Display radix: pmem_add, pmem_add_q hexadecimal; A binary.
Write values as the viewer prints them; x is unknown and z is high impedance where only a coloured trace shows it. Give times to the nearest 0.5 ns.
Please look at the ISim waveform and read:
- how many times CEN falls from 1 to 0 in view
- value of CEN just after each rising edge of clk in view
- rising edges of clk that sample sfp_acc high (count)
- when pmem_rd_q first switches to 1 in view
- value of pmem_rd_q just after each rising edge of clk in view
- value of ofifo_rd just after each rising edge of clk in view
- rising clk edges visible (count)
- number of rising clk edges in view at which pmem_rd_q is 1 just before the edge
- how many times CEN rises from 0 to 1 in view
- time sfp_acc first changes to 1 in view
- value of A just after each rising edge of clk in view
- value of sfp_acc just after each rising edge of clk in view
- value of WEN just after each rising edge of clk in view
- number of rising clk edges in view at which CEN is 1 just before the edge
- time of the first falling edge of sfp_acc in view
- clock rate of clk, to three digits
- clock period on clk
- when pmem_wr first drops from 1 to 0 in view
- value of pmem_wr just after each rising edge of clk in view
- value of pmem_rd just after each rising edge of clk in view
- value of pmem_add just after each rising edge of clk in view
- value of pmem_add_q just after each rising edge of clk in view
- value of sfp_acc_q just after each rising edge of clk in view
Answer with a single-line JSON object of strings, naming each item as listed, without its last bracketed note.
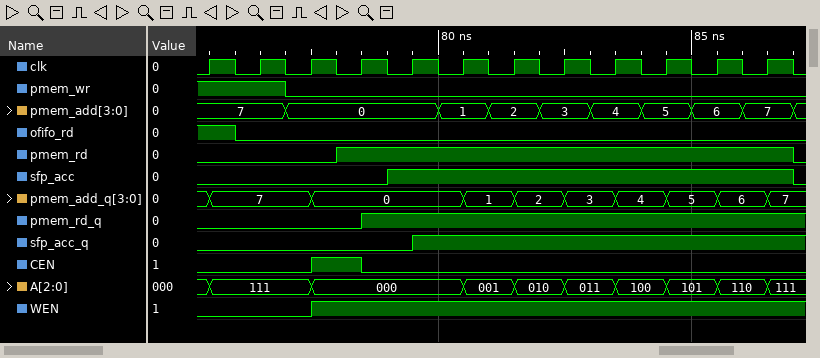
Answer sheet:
{"how many times CEN falls from 1 to 0 in view": "1", "value of CEN just after each rising edge of clk in view": "0 0 1 0 0 0 0 0 0 0 0 0", "rising edges of clk that sample sfp_acc high": "8", "when pmem_rd_q first switches to 1 in view": "78.5 ns", "value of pmem_rd_q just after each rising edge of clk in view": "0 0 0 1 1 1 1 1 1 1 1 1", "value of ofifo_rd just after each rising edge of clk in view": "1 0 0 0 0 0 0 0 0 0 0 0", "rising clk edges visible": "12", "number of rising clk edges in view at which pmem_rd_q is 1 just before the edge": "8", "how many times CEN rises from 0 to 1 in view": "1", "time sfp_acc first changes to 1 in view": "79 ns", "value of A just after each rising edge of clk in view": "111, 111, 000, 000, 000, 001, 010, 011, 100, 101, 110, 111", "value of sfp_acc just after each rising edge of clk in view": "0 0 0 0 1 1 1 1 1 1 1 1", "value of WEN just after each rising edge of clk in view": "0 0 1 1 1 1 1 1 1 1 1 1", "number of rising clk edges in view at which CEN is 1 just before the edge": "1", "time of the first falling edge of sfp_acc in view": "87 ns", "clock rate of clk, to three digits": "1.00 GHz", "clock period on clk": "1 ns", "when pmem_wr first drops from 1 to 0 in view": "77 ns", "value of pmem_wr just after each rising edge of clk in view": "1 1 0 0 0 0 0 0 0 0 0 0", "value of pmem_rd just after each rising edge of clk in view": "0 0 0 1 1 1 1 1 1 1 1 1", "value of pmem_add just after each rising edge of clk in view": "7, 7, 0, 0, 0, 1, 2, 3, 4, 5, 6, 7", "value of pmem_add_q just after each rising edge of clk in view": "7, 7, 0, 0, 0, 1, 2, 3, 4, 5, 6, 7", "value of sfp_acc_q just after each rising edge of clk in view": "0 0 0 0 1 1 1 1 1 1 1 1"}
